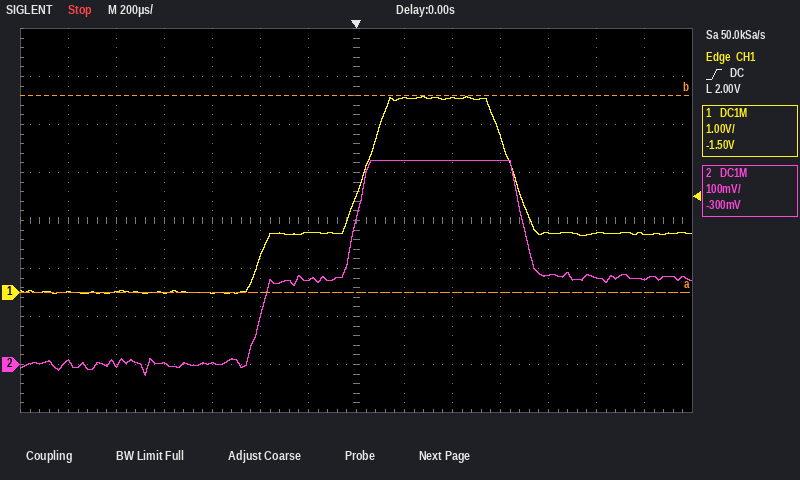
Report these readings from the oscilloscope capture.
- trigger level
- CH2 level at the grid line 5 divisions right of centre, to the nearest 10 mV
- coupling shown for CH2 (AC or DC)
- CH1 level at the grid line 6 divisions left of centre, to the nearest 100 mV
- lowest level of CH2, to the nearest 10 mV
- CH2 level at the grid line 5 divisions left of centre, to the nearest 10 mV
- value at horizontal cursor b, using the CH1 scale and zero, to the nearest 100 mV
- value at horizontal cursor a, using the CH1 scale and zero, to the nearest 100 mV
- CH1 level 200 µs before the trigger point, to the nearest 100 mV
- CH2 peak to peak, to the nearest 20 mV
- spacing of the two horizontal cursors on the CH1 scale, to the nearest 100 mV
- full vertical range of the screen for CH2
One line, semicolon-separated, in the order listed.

2.00 V; 180 mV; DC; 0.0 V; -20 mV; 0 mV; 4.1 V; 0.0 V; 1.2 V; 440 mV; 4.1 V; 800 mV
